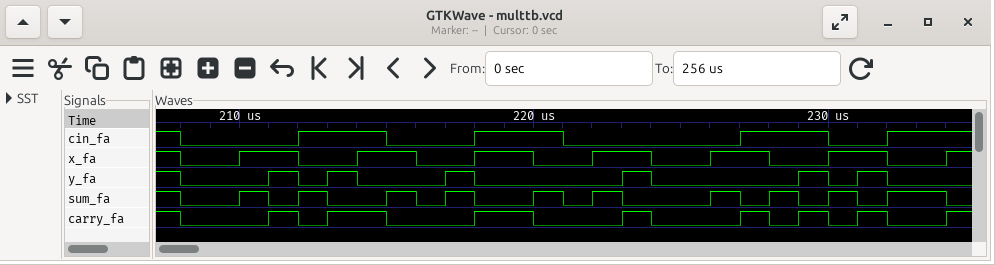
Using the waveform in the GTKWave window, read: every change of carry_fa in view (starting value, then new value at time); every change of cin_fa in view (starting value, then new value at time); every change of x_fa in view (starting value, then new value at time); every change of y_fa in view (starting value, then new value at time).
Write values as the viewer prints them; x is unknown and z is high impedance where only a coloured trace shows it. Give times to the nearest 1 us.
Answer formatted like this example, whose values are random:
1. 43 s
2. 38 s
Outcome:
1. 1, 0 at 208 us, 1 at 211 us, 0 at 212 us, 1 at 213 us, 0 at 215 us, 1 at 218 us, 0 at 220 us, 1 at 223 us, 0 at 224 us, 1 at 227 us, 0 at 228 us, 1 at 229 us, 0 at 230 us, 1 at 231 us, 0 at 232 us, 1 at 234 us
2. 1, 0 at 208 us, 1 at 212 us, 0 at 215 us, 1 at 218 us, 0 at 221 us, 1 at 227 us, 0 at 230 us, 1 at 232 us
3. 1, 0 at 208 us, 1 at 210 us, 0 at 212 us, 1 at 214 us, 0 at 216 us, 1 at 218 us, 0 at 220 us, 1 at 222 us, 0 at 224 us, 1 at 226 us, 0 at 228 us, 1 at 230 us, 0 at 232 us, 1 at 234 us
4. 1, 0 at 208 us, 1 at 211 us, 0 at 212 us, 1 at 213 us, 0 at 214 us, 1 at 217 us, 0 at 218 us, 1 at 223 us, 0 at 224 us, 1 at 229 us, 0 at 230 us, 1 at 231 us, 0 at 232 us
